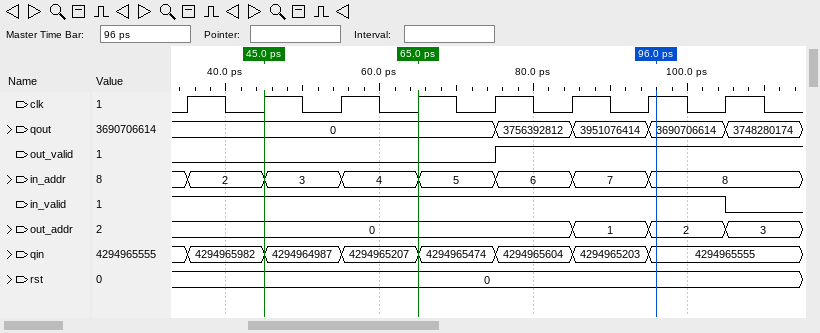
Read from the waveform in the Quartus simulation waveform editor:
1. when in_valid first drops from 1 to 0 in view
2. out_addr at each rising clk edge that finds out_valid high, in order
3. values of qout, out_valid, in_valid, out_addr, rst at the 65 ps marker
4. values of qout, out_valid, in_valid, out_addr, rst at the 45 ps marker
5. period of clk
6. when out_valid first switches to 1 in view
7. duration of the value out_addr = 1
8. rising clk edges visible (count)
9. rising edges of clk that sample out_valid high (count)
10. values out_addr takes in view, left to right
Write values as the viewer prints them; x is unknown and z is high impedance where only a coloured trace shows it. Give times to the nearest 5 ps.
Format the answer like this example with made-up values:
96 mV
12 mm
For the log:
105 ps
0, 1, 2
qout=0, out_valid=0, in_valid=1, out_addr=0, rst=0
qout=0, out_valid=0, in_valid=1, out_addr=0, rst=0
10 ps
75 ps
10 ps
8
3
0, 1, 2, 3
